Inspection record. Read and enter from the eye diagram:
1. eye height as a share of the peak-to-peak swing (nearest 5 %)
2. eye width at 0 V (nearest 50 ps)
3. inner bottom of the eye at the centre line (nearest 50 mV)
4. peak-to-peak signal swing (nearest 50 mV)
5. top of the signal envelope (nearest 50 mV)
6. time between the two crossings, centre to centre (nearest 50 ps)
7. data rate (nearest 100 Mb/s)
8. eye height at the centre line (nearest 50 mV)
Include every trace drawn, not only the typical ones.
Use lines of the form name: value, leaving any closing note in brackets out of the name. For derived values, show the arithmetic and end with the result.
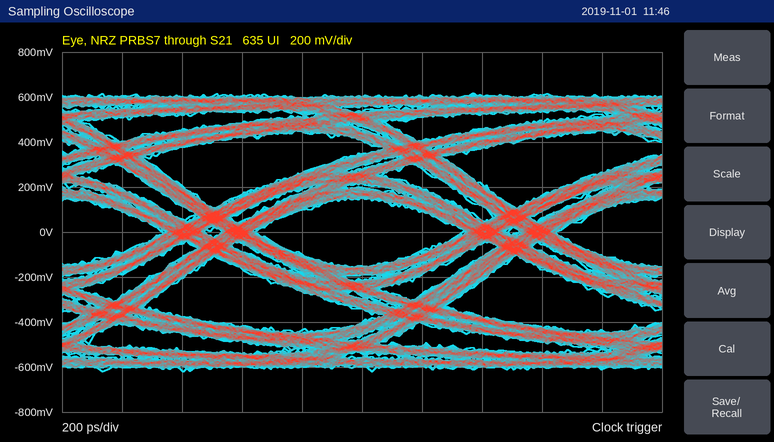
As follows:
eye height as a share of the peak-to-peak swing: 300 mV / 1.25 V ≈ 24.0 %, so 25 % to the nearest 5 %
eye width at 0 V: 700 ps
inner bottom of the eye at the centre line: -150 mV
peak-to-peak signal swing: 1.25 V
top of the signal envelope: 600 mV
time between the two crossings, centre to centre: 1.00 ns
data rate: 1.0 Gb/s
eye height at the centre line: 300 mV
